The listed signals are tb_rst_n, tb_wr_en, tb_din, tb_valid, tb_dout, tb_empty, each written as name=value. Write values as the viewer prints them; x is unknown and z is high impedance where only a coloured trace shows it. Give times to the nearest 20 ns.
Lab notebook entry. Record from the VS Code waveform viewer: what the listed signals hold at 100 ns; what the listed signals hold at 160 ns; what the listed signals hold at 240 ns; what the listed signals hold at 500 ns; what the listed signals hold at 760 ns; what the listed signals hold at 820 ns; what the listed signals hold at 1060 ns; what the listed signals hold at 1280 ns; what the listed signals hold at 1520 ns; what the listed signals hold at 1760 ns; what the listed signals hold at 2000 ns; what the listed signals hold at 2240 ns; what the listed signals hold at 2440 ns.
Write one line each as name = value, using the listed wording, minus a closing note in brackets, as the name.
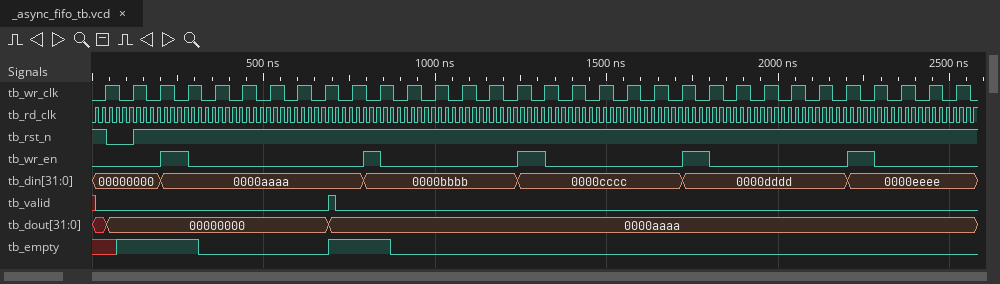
what the listed signals hold at 100 ns = tb_rst_n=0, tb_wr_en=0, tb_din=00000000, tb_valid=0, tb_dout=00000000, tb_empty=1
what the listed signals hold at 160 ns = tb_rst_n=1, tb_wr_en=0, tb_din=00000000, tb_valid=0, tb_dout=00000000, tb_empty=1
what the listed signals hold at 240 ns = tb_rst_n=1, tb_wr_en=1, tb_din=0000aaaa, tb_valid=0, tb_dout=00000000, tb_empty=1
what the listed signals hold at 500 ns = tb_rst_n=1, tb_wr_en=0, tb_din=0000aaaa, tb_valid=0, tb_dout=00000000, tb_empty=0
what the listed signals hold at 760 ns = tb_rst_n=1, tb_wr_en=0, tb_din=0000aaaa, tb_valid=0, tb_dout=0000aaaa, tb_empty=1
what the listed signals hold at 820 ns = tb_rst_n=1, tb_wr_en=1, tb_din=0000bbbb, tb_valid=0, tb_dout=0000aaaa, tb_empty=1
what the listed signals hold at 1060 ns = tb_rst_n=1, tb_wr_en=0, tb_din=0000bbbb, tb_valid=0, tb_dout=0000aaaa, tb_empty=0
what the listed signals hold at 1280 ns = tb_rst_n=1, tb_wr_en=1, tb_din=0000cccc, tb_valid=0, tb_dout=0000aaaa, tb_empty=0
what the listed signals hold at 1520 ns = tb_rst_n=1, tb_wr_en=0, tb_din=0000cccc, tb_valid=0, tb_dout=0000aaaa, tb_empty=0
what the listed signals hold at 1760 ns = tb_rst_n=1, tb_wr_en=1, tb_din=0000dddd, tb_valid=0, tb_dout=0000aaaa, tb_empty=0
what the listed signals hold at 2000 ns = tb_rst_n=1, tb_wr_en=0, tb_din=0000dddd, tb_valid=0, tb_dout=0000aaaa, tb_empty=0
what the listed signals hold at 2240 ns = tb_rst_n=1, tb_wr_en=1, tb_din=0000eeee, tb_valid=0, tb_dout=0000aaaa, tb_empty=0
what the listed signals hold at 2440 ns = tb_rst_n=1, tb_wr_en=0, tb_din=0000eeee, tb_valid=0, tb_dout=0000aaaa, tb_empty=0
